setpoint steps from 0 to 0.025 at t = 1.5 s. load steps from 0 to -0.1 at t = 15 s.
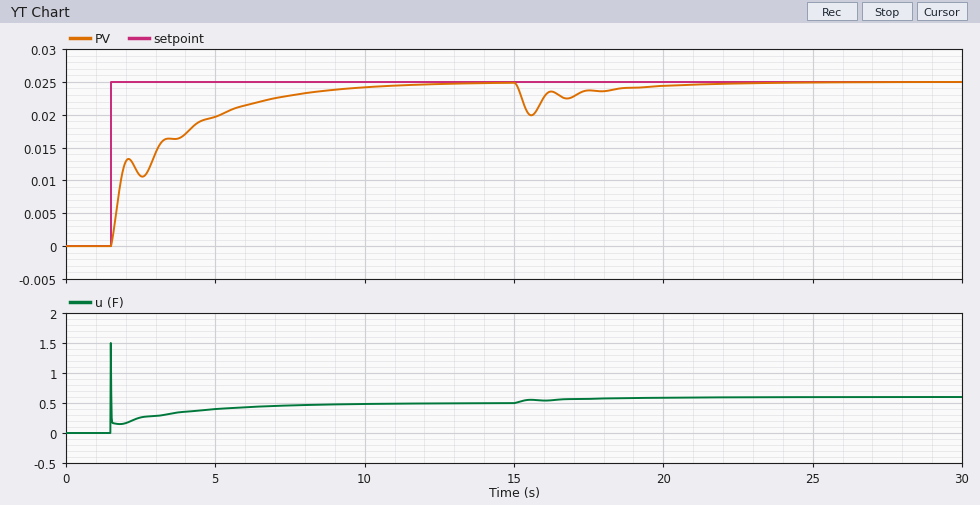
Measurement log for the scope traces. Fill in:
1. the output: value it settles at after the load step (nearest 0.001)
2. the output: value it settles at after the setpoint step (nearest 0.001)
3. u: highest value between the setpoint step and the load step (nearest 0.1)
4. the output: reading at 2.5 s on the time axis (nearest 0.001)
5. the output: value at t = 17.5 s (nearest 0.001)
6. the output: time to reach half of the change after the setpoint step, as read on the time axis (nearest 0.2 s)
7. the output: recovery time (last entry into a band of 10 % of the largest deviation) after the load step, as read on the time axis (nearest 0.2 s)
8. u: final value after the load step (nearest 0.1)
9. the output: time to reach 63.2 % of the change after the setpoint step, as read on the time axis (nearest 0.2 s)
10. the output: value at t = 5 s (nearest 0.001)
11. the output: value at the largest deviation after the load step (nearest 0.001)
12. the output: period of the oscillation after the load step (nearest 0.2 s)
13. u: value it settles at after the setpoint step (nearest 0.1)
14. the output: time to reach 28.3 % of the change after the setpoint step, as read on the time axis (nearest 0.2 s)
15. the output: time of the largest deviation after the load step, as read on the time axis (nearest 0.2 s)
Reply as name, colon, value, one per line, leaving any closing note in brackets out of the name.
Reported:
the output: value it settles at after the load step: 0.025
the output: value it settles at after the setpoint step: 0.025
u: highest value between the setpoint step and the load step: 1.5
the output: reading at 2.5 s on the time axis: 0.011
the output: value at t = 17.5 s: 0.024
the output: time to reach half of the change after the setpoint step, as read on the time axis: 2.0 s
the output: recovery time (last entry into a band of 10 % of the largest deviation) after the load step, as read on the time axis: 20.6 s
u: final value after the load step: 0.6
the output: time to reach 63.2 % of the change after the setpoint step, as read on the time axis: 3.2 s
the output: value at t = 5 s: 0.020
the output: value at the largest deviation after the load step: 0.020
the output: period of the oscillation after the load step: 1.2 s
u: value it settles at after the setpoint step: 0.5
the output: time to reach 28.3 % of the change after the setpoint step, as read on the time axis: 1.8 s
the output: time of the largest deviation after the load step, as read on the time axis: 15.6 s
